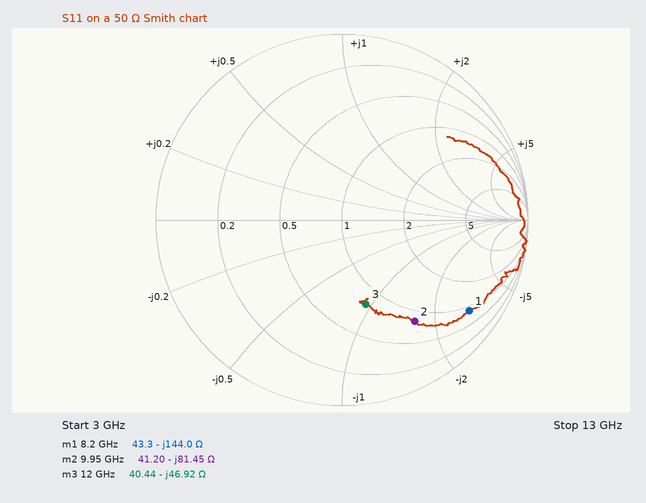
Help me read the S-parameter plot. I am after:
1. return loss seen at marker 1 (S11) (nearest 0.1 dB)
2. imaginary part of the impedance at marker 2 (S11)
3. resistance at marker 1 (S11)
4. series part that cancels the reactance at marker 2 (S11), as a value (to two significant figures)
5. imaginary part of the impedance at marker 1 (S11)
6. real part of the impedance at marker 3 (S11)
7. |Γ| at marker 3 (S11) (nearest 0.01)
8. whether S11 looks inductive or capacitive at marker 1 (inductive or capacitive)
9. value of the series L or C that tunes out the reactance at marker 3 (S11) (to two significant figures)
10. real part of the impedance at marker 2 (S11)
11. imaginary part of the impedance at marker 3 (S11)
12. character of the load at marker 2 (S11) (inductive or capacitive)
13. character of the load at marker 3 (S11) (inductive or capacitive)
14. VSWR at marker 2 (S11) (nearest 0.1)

1.5 dB
-81.45 Ω
43.3 Ω
1.3 nH
-144.0 Ω
40.44 Ω
0.47
capacitive
620 pH
41.20 Ω
-46.92 Ω
capacitive
capacitive
5.1
